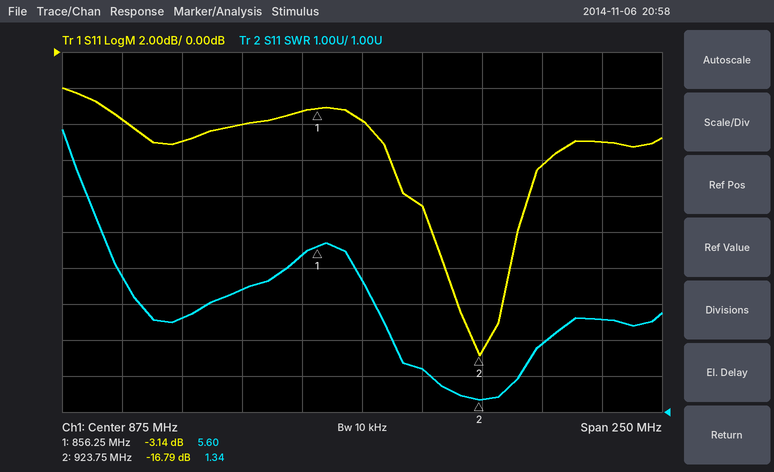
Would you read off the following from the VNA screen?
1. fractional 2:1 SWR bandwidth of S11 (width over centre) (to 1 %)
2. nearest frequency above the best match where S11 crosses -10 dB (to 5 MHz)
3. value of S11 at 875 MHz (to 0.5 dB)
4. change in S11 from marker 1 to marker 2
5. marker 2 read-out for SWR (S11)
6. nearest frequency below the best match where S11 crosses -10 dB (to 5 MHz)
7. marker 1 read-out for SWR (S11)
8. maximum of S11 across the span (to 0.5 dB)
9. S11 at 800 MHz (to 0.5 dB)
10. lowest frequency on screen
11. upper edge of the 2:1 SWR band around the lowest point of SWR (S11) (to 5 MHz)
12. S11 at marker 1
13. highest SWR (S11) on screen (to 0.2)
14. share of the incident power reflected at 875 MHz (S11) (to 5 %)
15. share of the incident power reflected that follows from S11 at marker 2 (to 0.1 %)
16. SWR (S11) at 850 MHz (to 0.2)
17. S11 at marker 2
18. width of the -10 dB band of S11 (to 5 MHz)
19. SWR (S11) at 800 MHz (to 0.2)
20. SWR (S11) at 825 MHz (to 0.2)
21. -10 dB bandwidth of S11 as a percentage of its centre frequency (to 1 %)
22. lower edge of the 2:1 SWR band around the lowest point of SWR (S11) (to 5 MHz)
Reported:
4 %
940 MHz
-4.0 dB
-13.65 dB
1.34
905 MHz
5.60
-2.0 dB
-5.0 dB
750 MHz
940 MHz
-3.14 dB
8.8
40 %
2.1 %
5.4
-16.79 dB
35 MHz
3.6
4.4
4 %
905 MHz
